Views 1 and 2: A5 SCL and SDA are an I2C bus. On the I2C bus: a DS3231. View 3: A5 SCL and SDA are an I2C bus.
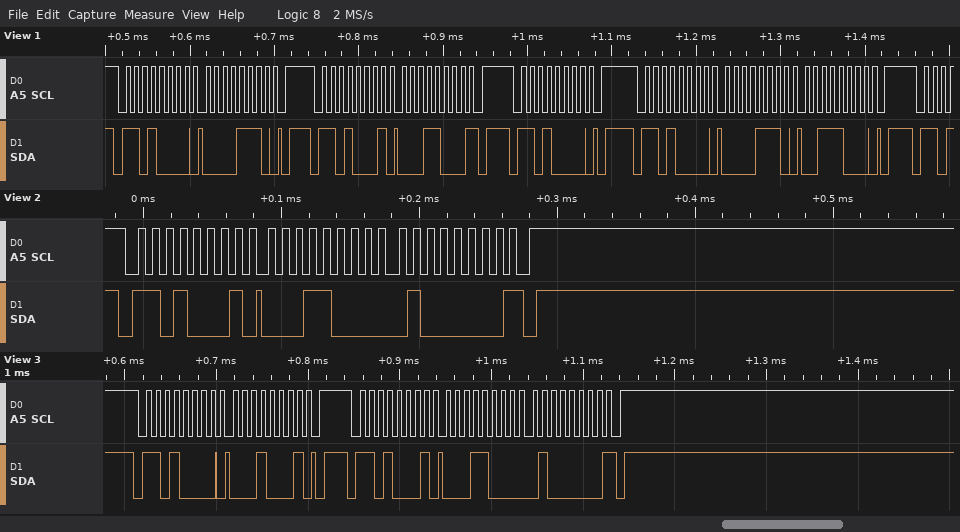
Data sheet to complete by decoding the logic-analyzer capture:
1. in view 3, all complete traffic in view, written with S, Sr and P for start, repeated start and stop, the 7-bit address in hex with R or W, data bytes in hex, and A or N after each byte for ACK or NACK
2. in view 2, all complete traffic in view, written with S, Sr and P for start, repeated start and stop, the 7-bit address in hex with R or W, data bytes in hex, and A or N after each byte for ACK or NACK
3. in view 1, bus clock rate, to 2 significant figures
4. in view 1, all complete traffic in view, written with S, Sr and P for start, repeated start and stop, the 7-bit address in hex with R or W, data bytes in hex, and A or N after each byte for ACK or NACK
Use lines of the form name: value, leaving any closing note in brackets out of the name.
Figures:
in view 3, all complete traffic in view, written with S, Sr and P for start, repeated start and stop, the 7-bit address in hex with R or W, data bytes in hex, and A or N after each byte for ACK or NACK: S 68W A 11 A P S 68R A 18 A 40 N P
in view 2, all complete traffic in view, written with S, Sr and P for start, repeated start and stop, the 7-bit address in hex with R or W, data bytes in hex, and A or N after each byte for ACK or NACK: S 68R A 18 A 40 N P
in view 1, bus clock rate, to 2 significant figures: 100 kHz
in view 1, all complete traffic in view, written with S, Sr and P for start, repeated start and stop, the 7-bit address in hex with R or W, data bytes in hex, and A or N after each byte for ACK or NACK: S 68W A 0E A P S 68R A 18 N P S 68W A P S 68W A 0E A 38 A P
